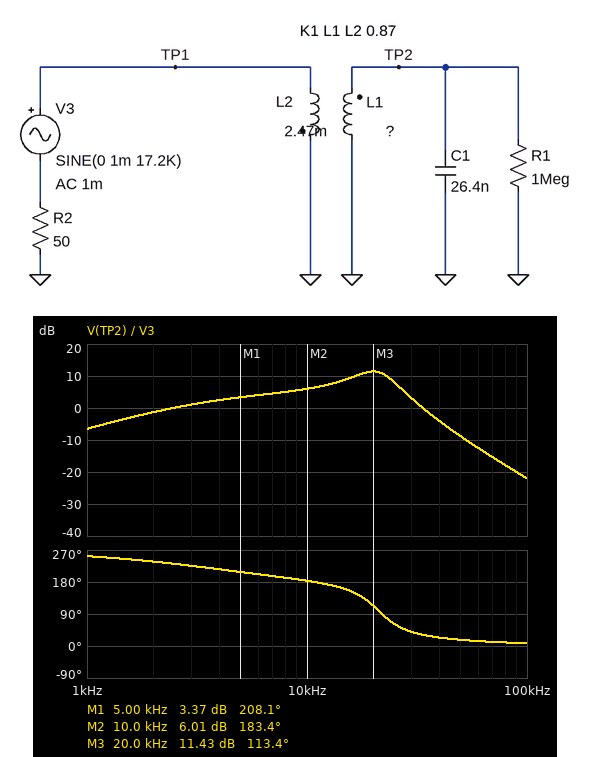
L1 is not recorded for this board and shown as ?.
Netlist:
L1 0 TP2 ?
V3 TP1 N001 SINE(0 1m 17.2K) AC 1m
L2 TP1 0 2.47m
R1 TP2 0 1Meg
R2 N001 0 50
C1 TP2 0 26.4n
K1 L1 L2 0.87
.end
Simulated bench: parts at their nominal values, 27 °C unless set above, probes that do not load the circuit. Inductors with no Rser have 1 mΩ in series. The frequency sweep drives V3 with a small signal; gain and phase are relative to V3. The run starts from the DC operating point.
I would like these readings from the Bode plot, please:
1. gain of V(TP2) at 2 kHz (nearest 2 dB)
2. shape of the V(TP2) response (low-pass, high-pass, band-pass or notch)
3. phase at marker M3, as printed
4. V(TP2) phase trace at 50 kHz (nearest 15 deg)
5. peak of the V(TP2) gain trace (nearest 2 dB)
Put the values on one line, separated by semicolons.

-2 dB; band-pass; 113.4 deg; 15 deg; 12 dB
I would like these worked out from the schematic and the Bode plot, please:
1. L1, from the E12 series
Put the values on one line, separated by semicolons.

8.2 mH
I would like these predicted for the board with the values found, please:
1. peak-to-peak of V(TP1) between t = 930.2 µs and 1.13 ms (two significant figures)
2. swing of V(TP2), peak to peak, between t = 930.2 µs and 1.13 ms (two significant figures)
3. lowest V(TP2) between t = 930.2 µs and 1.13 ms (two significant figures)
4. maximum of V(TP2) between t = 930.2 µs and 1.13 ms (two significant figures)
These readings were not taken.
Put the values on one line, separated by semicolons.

1.6 mV; 6.6 mV; -3.3 mV; 3.3 mV
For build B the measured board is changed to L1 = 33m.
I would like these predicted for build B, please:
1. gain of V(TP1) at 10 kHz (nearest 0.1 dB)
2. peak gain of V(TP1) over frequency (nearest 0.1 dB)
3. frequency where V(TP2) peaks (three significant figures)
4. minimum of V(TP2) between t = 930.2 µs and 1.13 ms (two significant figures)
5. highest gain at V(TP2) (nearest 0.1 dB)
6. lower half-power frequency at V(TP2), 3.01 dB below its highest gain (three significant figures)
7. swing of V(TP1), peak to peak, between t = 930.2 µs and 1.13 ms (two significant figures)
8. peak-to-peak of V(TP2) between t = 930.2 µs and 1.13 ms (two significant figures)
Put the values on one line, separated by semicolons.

-13.8 dB; 0 dB; 7.46 kHz; -1.4 mV; 13.6 dB; 3.99 kHz; 1.3 mV; 2.8 mV
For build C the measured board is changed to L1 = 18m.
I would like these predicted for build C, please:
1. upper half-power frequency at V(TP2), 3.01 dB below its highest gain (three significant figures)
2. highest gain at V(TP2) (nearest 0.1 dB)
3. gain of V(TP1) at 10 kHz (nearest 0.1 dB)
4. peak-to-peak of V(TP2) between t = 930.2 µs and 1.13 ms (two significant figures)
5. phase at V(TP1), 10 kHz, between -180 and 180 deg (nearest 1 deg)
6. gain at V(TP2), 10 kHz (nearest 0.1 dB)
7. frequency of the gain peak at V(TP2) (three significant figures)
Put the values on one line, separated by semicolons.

16.2 kHz; 12.3 dB; -1.0 dB; 5.1 mV; -27 deg; 11.7 dB; 12.0 kHz
